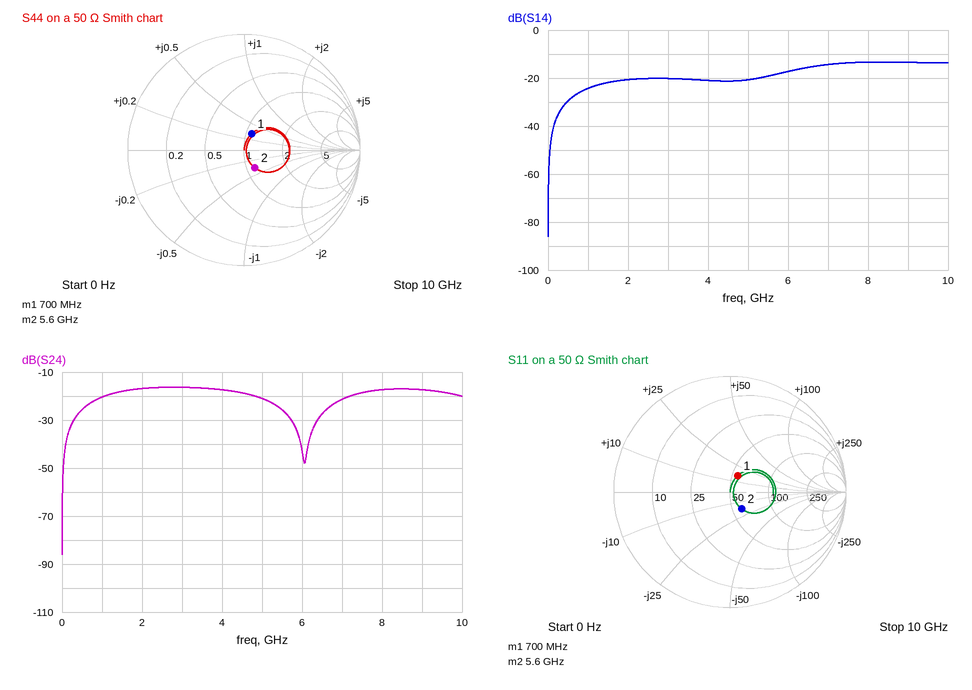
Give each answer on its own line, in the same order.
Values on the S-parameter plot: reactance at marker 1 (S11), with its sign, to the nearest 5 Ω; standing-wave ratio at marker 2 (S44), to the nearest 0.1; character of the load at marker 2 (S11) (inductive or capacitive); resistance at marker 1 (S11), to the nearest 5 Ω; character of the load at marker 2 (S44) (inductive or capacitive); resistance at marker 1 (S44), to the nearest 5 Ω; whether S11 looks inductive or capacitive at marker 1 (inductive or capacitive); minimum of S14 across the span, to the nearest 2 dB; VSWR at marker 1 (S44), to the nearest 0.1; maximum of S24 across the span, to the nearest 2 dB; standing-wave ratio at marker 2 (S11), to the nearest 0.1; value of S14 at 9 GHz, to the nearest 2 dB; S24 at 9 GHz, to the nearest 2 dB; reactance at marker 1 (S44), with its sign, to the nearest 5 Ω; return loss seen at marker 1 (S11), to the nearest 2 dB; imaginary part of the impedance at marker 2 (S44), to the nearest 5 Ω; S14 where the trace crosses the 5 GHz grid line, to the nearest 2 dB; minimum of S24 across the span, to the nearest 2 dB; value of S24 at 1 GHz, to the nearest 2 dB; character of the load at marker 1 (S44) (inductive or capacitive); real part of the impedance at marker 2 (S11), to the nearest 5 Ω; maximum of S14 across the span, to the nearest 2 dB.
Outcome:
+15 Ω
1.4
capacitive
55 Ω
capacitive
55 Ω
inductive
-86 dB
1.4
-16 dB
1.4
-14 dB
-18 dB
+15 Ω
16 dB
-20 Ω
-20 dB
-86 dB
-20 dB
inductive
60 Ω
-14 dB
